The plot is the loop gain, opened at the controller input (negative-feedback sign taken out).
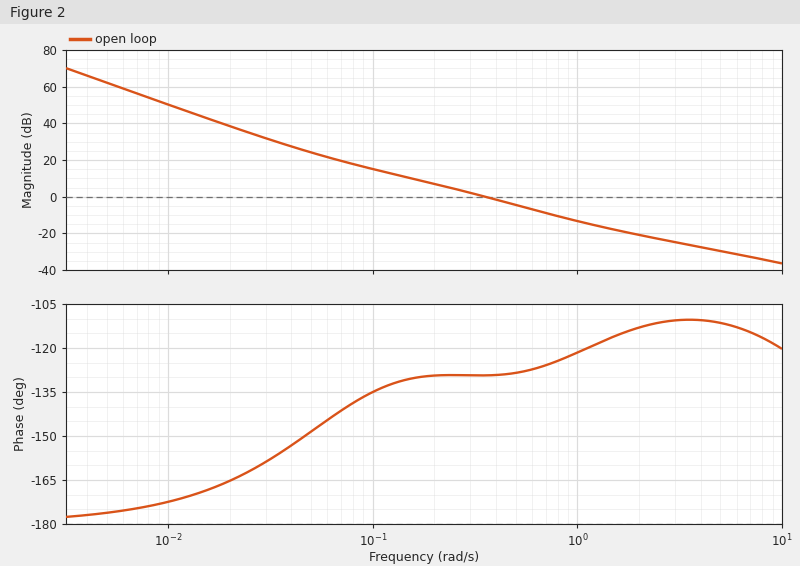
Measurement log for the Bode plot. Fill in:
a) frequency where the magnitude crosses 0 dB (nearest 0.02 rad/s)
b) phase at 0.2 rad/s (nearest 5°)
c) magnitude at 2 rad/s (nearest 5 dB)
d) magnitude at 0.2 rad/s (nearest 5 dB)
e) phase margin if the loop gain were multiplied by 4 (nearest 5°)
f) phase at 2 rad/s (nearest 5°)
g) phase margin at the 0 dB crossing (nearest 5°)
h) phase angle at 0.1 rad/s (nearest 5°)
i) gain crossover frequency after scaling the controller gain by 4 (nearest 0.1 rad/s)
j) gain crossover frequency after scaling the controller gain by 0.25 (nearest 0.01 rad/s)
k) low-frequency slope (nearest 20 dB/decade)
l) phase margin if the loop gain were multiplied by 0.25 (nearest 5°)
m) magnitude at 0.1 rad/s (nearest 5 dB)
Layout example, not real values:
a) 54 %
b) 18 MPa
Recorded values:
a) 0.36 rad/s
b) -130°
c) -20 dB
d) 5 dB
e) 55°
f) -115°
g) 50°
h) -135°
i) 0.9 rad/s
j) 0.13 rad/s
k) -40 dB/decade
l) 50°
m) 15 dB
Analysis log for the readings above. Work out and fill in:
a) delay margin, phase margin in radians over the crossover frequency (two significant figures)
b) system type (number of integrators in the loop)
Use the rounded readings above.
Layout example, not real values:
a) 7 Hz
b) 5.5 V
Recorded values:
a) 2.4 s
b) 2
